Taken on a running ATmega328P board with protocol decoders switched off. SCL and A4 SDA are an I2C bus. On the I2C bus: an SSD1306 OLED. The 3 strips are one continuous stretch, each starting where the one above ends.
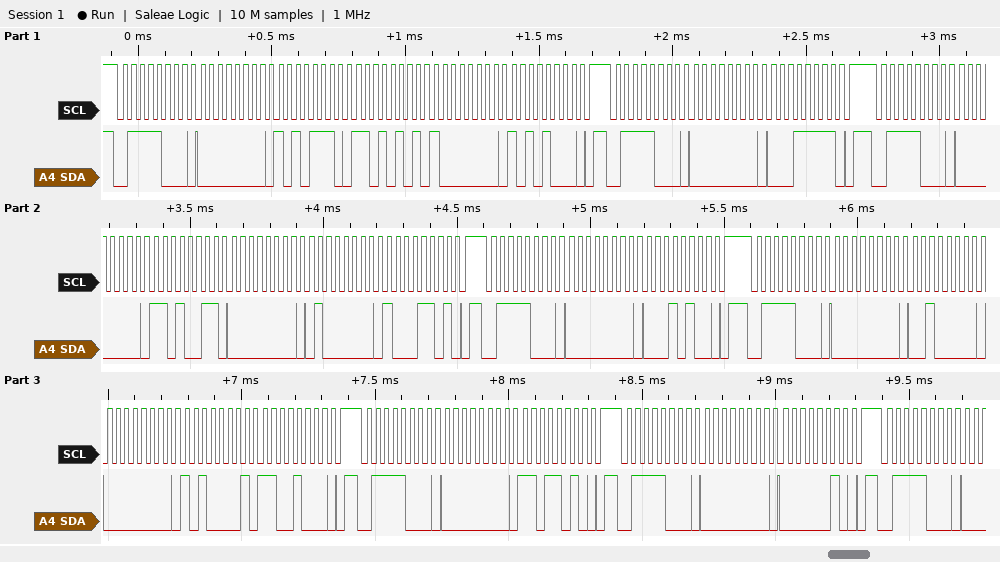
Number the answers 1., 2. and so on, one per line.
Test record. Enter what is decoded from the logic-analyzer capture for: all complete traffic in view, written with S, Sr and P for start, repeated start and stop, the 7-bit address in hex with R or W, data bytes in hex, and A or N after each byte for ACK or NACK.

1. S 3CW A 00 A AE A D5 A 80 A A8 A P S 3CW A 00 A 1F A P S 3CW A 00 A D3 A 00 A 40 A 8D A P S 3CW A 00 A 14 A P S 3CW A 00 A 20 A 00 A A1 A C8 A P S 3CW A 00 A DA A P S 3CW A 00 A 02 A P S 3CW A
